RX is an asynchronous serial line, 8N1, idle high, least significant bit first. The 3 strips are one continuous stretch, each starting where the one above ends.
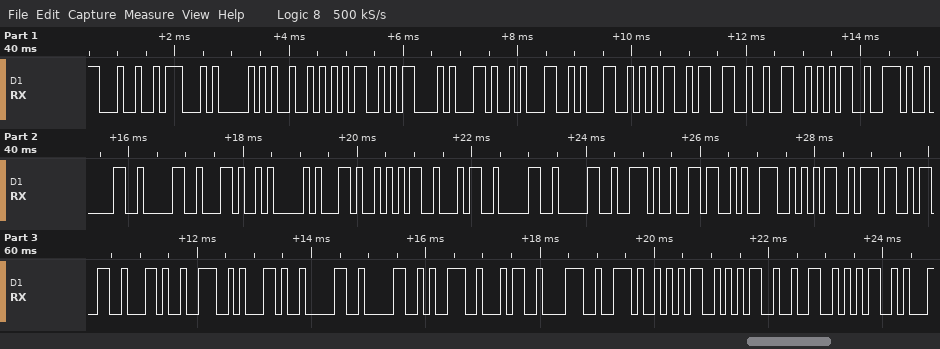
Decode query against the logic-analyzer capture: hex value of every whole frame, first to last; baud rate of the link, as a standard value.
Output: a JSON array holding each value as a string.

["24 47 50 52 4D 43 2C 31 31 35 33 32 35 2E 30 30 2C 41 2C 35 34 30 30 2E 36 39 35 37 33 2C 4E 2C 30 30 39 34 38 2E 35 35 32 35", "9600 baud"]
